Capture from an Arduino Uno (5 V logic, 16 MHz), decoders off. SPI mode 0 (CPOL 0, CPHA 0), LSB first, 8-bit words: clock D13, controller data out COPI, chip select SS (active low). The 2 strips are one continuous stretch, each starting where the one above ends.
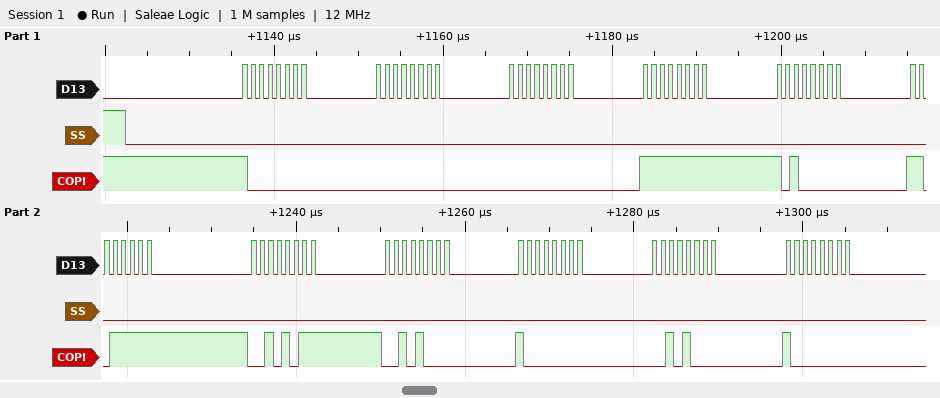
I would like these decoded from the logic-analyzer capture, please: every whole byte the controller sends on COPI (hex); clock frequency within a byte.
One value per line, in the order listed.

01 00 00 FF 05 FB D4 14 01 14 01
1 MHz
